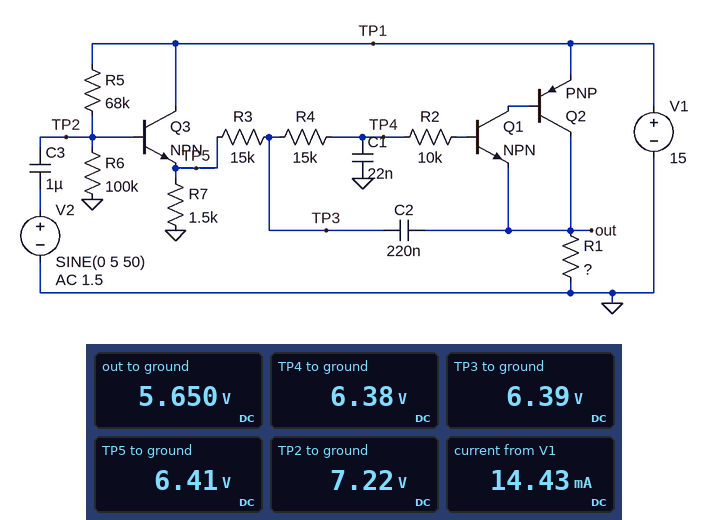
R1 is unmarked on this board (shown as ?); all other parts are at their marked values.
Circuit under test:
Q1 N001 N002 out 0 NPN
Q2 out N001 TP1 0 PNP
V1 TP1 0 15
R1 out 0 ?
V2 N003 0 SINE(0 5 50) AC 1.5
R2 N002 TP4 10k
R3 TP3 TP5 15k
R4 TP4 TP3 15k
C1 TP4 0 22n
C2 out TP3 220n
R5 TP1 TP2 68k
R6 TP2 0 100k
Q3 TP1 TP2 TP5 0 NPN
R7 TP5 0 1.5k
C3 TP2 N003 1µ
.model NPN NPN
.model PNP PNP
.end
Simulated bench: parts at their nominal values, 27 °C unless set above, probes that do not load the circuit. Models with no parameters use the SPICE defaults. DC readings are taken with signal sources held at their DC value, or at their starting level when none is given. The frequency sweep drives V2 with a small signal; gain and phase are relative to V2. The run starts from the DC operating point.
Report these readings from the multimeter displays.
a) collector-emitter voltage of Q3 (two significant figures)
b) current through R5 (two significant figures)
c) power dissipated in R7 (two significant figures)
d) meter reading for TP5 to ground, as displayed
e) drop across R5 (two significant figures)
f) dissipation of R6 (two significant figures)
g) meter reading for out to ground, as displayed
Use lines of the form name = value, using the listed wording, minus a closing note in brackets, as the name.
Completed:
collector-emitter voltage of Q3 = 8.6 V
current through R5 = 110 µA
power dissipated in R7 = 27 mW
meter reading for TP5 to ground, as displayed = 6.41 V
drop across R5 = 7.8 V
dissipation of R6 = 520 µW
meter reading for out to ground, as displayed = 5.650 V
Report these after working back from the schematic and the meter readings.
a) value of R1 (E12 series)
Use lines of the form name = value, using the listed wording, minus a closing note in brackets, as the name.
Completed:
value of R1 = 560 Ω
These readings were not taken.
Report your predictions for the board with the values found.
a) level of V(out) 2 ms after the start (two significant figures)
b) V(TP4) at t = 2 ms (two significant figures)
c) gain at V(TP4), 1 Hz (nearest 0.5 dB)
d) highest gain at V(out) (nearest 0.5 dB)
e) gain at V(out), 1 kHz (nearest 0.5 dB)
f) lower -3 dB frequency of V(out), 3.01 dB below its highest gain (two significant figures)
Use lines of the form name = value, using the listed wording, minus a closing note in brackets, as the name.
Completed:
level of V(out) 2 ms after the start = 6.8 V
V(TP4) at t = 2 ms = 7.5 V
gain at V(TP4), 1 Hz = -14.0 dB
highest gain at V(out) = 4.0 dB
gain at V(out), 1 kHz = -32.5 dB
lower -3 dB frequency of V(out), 3.01 dB below its highest gain = 61 Hz
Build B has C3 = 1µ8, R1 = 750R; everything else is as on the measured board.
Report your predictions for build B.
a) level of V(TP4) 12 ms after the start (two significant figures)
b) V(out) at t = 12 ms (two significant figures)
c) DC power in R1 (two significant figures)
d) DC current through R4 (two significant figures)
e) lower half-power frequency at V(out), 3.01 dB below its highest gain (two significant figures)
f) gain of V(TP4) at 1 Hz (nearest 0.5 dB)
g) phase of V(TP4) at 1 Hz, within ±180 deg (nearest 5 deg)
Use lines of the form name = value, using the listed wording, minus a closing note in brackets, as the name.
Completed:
level of V(TP4) 12 ms after the start = 3.9 V
V(out) at t = 12 ms = 3.2 V
DC power in R1 = 43 mW
DC current through R4 = 750 nA
lower half-power frequency at V(out), 3.01 dB below its highest gain = 62 Hz
gain of V(TP4) at 1 Hz = -9.5 dB
phase of V(TP4) at 1 Hz, within ±180 deg = 70 deg
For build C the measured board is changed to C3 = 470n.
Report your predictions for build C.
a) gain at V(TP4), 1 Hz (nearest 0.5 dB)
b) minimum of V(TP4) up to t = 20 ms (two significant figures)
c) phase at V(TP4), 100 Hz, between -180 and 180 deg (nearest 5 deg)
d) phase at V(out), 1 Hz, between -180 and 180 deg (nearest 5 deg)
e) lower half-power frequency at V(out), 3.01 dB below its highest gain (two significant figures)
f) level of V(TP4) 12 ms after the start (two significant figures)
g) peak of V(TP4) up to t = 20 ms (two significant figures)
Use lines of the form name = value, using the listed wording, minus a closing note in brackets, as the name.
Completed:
gain at V(TP4), 1 Hz = -20.5 dB
minimum of V(TP4) up to t = 20 ms = 820 mV
phase at V(TP4), 100 Hz, between -180 and 180 deg = -30 deg
phase at V(out), 1 Hz, between -180 and 180 deg = 85 deg
lower half-power frequency at V(out), 3.01 dB below its highest gain = 63 Hz
level of V(TP4) 12 ms after the start = 3.0 V
peak of V(TP4) up to t = 20 ms = 11 V
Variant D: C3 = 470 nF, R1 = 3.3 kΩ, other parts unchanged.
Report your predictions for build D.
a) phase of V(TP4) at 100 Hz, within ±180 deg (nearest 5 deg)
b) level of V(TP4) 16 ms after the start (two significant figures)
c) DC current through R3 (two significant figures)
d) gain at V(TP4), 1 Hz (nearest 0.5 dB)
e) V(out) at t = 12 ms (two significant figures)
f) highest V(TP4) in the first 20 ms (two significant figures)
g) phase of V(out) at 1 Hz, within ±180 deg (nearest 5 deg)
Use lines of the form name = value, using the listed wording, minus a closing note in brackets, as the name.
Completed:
phase of V(TP4) at 100 Hz, within ±180 deg = -30 deg
level of V(TP4) 16 ms after the start = 1.0 V
DC current through R3 = 170 nA
gain at V(TP4), 1 Hz = -20.5 dB
V(out) at t = 12 ms = 2.3 V
highest V(TP4) in the first 20 ms = 11 V
phase of V(out) at 1 Hz, within ±180 deg = 85 deg
